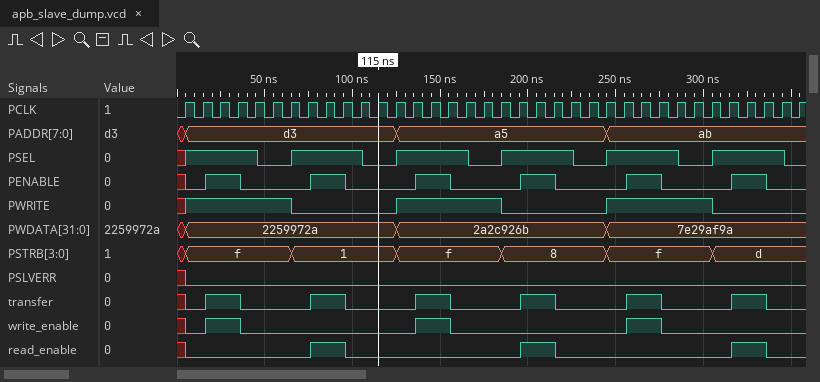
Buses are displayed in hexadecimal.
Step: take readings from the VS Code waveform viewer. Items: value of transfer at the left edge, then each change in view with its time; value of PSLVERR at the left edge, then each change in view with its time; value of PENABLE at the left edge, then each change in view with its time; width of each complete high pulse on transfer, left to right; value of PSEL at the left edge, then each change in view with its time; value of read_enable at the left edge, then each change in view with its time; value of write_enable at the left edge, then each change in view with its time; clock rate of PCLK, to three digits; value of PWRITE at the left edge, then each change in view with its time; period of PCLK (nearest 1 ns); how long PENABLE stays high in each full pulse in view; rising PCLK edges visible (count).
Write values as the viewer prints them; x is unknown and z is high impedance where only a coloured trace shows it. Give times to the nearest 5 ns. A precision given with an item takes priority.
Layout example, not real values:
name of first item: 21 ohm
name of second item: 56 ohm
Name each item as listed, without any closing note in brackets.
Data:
value of transfer at the left edge, then each change in view with its time: x, 0 at 5 ns, 1 at 15 ns, 0 at 35 ns, 1 at 75 ns, 0 at 95 ns, 1 at 135 ns, 0 at 155 ns, 1 at 195 ns, 0 at 215 ns, 1 at 255 ns, 0 at 275 ns, 1 at 315 ns, 0 at 335 ns
value of PSLVERR at the left edge, then each change in view with its time: x, 0 at 5 ns
value of PENABLE at the left edge, then each change in view with its time: x, 0 at 5 ns, 1 at 15 ns, 0 at 35 ns, 1 at 75 ns, 0 at 95 ns, 1 at 135 ns, 0 at 155 ns, 1 at 195 ns, 0 at 215 ns, 1 at 255 ns, 0 at 275 ns, 1 at 315 ns, 0 at 335 ns
width of each complete high pulse on transfer, left to right: 20 ns, 20 ns, 20 ns, 20 ns, 20 ns, 20 ns
value of PSEL at the left edge, then each change in view with its time: x, 1 at 5 ns, 0 at 45 ns, 1 at 65 ns, 0 at 105 ns, 1 at 125 ns, 0 at 165 ns, 1 at 185 ns, 0 at 225 ns, 1 at 245 ns, 0 at 285 ns, 1 at 305 ns, 0 at 345 ns
value of read_enable at the left edge, then each change in view with its time: x, 0 at 5 ns, 1 at 75 ns, 0 at 95 ns, 1 at 195 ns, 0 at 215 ns, 1 at 315 ns, 0 at 335 ns
value of write_enable at the left edge, then each change in view with its time: x, 0 at 5 ns, 1 at 15 ns, 0 at 35 ns, 1 at 135 ns, 0 at 155 ns, 1 at 255 ns, 0 at 275 ns
clock rate of PCLK, to three digits: 100 MHz
value of PWRITE at the left edge, then each change in view with its time: x, 1 at 5 ns, 0 at 65 ns, 1 at 125 ns, 0 at 185 ns, 1 at 245 ns, 0 at 305 ns
period of PCLK: 10 ns
how long PENABLE stays high in each full pulse in view: 20 ns, 20 ns, 20 ns, 20 ns, 20 ns, 20 ns
rising PCLK edges visible: 36
